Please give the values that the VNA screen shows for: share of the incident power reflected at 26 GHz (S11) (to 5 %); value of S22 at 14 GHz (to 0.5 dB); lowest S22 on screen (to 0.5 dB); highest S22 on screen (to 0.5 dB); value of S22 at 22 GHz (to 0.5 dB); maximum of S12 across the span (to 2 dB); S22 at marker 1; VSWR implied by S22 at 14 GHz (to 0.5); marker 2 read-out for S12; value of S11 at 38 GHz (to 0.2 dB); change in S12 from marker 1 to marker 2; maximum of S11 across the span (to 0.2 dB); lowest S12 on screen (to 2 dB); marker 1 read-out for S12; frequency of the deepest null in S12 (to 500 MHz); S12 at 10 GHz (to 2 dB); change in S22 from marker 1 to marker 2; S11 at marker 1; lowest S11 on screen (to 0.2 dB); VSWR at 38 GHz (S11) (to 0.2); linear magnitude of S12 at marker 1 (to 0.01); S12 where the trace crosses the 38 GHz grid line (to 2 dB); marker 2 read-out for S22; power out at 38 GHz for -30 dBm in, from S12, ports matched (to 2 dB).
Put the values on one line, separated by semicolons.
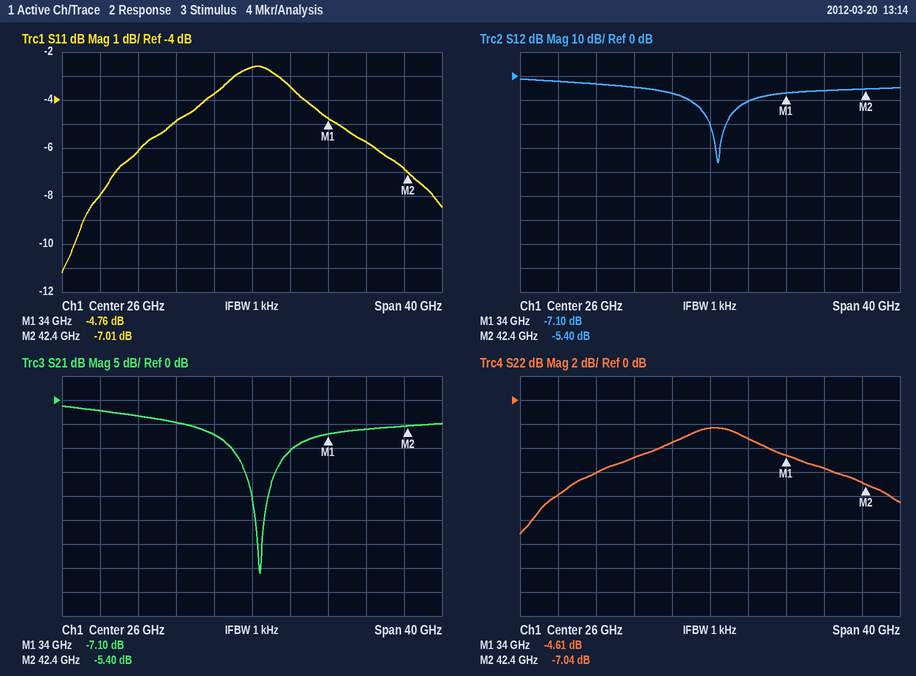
55 %; -6.0 dB; -11.0 dB; -2.5 dB; -3.5 dB; -2 dB; -4.61 dB; 3.0; -5.40 dB; -5.8 dB; 1.70 dB; -2.6 dB; -36 dB; -7.10 dB; 27.0 GHz; -2 dB; -2.43 dB; -4.76 dB; -11.2 dB; 3.2; 0.44; -6 dB; -7.04 dB; -36 dBm
